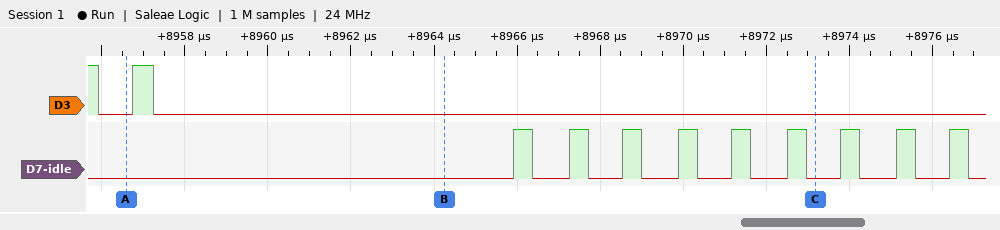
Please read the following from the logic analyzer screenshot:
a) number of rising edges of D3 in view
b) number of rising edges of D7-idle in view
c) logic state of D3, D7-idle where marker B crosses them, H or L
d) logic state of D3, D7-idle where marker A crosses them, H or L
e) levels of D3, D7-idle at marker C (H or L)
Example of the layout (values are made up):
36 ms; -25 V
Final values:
1; 9; D3=L, D7-idle=L; D3=L, D7-idle=L; D3=L, D7-idle=L
